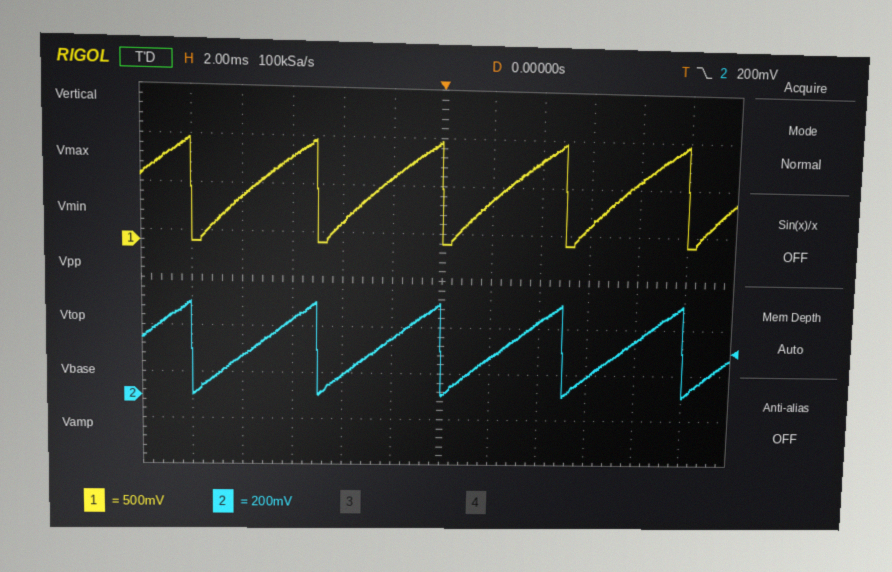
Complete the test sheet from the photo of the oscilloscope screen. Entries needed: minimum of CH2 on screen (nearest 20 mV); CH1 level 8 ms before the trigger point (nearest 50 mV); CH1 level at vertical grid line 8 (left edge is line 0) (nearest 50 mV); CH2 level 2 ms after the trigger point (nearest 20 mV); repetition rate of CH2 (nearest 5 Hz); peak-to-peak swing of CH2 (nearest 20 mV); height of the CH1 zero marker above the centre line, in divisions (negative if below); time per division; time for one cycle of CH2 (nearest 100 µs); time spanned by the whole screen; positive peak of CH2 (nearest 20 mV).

0 mV
450 mV
900 mV
180 mV
200 Hz
400 mV
+0.8 div
2 ms
5.0 ms
24 ms
400 mV
